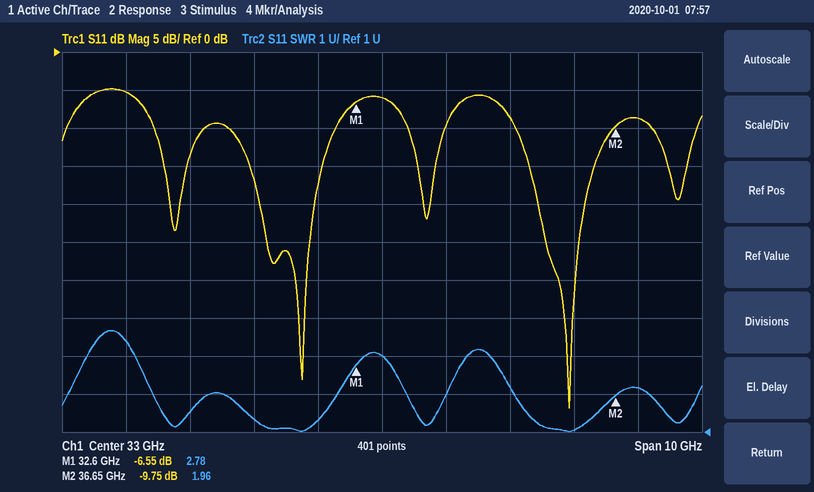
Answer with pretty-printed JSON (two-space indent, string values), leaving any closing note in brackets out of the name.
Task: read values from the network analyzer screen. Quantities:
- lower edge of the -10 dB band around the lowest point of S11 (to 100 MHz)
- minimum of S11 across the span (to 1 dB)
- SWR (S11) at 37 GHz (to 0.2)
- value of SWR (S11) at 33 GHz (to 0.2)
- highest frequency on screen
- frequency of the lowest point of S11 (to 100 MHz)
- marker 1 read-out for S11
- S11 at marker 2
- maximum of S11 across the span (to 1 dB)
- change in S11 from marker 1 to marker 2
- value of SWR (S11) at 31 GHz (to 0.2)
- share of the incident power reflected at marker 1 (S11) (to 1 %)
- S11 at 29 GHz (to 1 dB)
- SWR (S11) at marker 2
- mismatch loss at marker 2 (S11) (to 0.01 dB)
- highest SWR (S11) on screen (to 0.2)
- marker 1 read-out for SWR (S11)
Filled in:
{
  "lower edge of the -10 dB band around the lowest point of S11": "35.1 GHz",
  "minimum of S11 across the span": "-47 dB",
  "SWR (S11) at 37 GHz": "2.2",
  "value of SWR (S11) at 33 GHz": "3.0",
  "highest frequency on screen": "38 GHz",
  "frequency of the lowest point of S11": "35.9 GHz",
  "marker 1 read-out for S11": "-6.55 dB",
  "S11 at marker 2": "-9.75 dB",
  "maximum of S11 across the span": "-5 dB",
  "change in S11 from marker 1 to marker 2": "-3.20 dB",
  "value of SWR (S11) at 31 GHz": "1.4",
  "share of the incident power reflected at marker 1 (S11)": "22 %",
  "S11 at 29 GHz": "-5 dB",
  "SWR (S11) at marker 2": "1.96",
  "mismatch loss at marker 2 (S11)": "0.49 dB",
  "highest SWR (S11) on screen": "3.6",
  "marker 1 read-out for SWR": "2.78"
}
